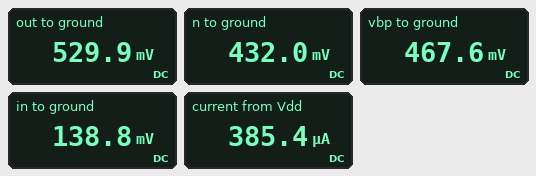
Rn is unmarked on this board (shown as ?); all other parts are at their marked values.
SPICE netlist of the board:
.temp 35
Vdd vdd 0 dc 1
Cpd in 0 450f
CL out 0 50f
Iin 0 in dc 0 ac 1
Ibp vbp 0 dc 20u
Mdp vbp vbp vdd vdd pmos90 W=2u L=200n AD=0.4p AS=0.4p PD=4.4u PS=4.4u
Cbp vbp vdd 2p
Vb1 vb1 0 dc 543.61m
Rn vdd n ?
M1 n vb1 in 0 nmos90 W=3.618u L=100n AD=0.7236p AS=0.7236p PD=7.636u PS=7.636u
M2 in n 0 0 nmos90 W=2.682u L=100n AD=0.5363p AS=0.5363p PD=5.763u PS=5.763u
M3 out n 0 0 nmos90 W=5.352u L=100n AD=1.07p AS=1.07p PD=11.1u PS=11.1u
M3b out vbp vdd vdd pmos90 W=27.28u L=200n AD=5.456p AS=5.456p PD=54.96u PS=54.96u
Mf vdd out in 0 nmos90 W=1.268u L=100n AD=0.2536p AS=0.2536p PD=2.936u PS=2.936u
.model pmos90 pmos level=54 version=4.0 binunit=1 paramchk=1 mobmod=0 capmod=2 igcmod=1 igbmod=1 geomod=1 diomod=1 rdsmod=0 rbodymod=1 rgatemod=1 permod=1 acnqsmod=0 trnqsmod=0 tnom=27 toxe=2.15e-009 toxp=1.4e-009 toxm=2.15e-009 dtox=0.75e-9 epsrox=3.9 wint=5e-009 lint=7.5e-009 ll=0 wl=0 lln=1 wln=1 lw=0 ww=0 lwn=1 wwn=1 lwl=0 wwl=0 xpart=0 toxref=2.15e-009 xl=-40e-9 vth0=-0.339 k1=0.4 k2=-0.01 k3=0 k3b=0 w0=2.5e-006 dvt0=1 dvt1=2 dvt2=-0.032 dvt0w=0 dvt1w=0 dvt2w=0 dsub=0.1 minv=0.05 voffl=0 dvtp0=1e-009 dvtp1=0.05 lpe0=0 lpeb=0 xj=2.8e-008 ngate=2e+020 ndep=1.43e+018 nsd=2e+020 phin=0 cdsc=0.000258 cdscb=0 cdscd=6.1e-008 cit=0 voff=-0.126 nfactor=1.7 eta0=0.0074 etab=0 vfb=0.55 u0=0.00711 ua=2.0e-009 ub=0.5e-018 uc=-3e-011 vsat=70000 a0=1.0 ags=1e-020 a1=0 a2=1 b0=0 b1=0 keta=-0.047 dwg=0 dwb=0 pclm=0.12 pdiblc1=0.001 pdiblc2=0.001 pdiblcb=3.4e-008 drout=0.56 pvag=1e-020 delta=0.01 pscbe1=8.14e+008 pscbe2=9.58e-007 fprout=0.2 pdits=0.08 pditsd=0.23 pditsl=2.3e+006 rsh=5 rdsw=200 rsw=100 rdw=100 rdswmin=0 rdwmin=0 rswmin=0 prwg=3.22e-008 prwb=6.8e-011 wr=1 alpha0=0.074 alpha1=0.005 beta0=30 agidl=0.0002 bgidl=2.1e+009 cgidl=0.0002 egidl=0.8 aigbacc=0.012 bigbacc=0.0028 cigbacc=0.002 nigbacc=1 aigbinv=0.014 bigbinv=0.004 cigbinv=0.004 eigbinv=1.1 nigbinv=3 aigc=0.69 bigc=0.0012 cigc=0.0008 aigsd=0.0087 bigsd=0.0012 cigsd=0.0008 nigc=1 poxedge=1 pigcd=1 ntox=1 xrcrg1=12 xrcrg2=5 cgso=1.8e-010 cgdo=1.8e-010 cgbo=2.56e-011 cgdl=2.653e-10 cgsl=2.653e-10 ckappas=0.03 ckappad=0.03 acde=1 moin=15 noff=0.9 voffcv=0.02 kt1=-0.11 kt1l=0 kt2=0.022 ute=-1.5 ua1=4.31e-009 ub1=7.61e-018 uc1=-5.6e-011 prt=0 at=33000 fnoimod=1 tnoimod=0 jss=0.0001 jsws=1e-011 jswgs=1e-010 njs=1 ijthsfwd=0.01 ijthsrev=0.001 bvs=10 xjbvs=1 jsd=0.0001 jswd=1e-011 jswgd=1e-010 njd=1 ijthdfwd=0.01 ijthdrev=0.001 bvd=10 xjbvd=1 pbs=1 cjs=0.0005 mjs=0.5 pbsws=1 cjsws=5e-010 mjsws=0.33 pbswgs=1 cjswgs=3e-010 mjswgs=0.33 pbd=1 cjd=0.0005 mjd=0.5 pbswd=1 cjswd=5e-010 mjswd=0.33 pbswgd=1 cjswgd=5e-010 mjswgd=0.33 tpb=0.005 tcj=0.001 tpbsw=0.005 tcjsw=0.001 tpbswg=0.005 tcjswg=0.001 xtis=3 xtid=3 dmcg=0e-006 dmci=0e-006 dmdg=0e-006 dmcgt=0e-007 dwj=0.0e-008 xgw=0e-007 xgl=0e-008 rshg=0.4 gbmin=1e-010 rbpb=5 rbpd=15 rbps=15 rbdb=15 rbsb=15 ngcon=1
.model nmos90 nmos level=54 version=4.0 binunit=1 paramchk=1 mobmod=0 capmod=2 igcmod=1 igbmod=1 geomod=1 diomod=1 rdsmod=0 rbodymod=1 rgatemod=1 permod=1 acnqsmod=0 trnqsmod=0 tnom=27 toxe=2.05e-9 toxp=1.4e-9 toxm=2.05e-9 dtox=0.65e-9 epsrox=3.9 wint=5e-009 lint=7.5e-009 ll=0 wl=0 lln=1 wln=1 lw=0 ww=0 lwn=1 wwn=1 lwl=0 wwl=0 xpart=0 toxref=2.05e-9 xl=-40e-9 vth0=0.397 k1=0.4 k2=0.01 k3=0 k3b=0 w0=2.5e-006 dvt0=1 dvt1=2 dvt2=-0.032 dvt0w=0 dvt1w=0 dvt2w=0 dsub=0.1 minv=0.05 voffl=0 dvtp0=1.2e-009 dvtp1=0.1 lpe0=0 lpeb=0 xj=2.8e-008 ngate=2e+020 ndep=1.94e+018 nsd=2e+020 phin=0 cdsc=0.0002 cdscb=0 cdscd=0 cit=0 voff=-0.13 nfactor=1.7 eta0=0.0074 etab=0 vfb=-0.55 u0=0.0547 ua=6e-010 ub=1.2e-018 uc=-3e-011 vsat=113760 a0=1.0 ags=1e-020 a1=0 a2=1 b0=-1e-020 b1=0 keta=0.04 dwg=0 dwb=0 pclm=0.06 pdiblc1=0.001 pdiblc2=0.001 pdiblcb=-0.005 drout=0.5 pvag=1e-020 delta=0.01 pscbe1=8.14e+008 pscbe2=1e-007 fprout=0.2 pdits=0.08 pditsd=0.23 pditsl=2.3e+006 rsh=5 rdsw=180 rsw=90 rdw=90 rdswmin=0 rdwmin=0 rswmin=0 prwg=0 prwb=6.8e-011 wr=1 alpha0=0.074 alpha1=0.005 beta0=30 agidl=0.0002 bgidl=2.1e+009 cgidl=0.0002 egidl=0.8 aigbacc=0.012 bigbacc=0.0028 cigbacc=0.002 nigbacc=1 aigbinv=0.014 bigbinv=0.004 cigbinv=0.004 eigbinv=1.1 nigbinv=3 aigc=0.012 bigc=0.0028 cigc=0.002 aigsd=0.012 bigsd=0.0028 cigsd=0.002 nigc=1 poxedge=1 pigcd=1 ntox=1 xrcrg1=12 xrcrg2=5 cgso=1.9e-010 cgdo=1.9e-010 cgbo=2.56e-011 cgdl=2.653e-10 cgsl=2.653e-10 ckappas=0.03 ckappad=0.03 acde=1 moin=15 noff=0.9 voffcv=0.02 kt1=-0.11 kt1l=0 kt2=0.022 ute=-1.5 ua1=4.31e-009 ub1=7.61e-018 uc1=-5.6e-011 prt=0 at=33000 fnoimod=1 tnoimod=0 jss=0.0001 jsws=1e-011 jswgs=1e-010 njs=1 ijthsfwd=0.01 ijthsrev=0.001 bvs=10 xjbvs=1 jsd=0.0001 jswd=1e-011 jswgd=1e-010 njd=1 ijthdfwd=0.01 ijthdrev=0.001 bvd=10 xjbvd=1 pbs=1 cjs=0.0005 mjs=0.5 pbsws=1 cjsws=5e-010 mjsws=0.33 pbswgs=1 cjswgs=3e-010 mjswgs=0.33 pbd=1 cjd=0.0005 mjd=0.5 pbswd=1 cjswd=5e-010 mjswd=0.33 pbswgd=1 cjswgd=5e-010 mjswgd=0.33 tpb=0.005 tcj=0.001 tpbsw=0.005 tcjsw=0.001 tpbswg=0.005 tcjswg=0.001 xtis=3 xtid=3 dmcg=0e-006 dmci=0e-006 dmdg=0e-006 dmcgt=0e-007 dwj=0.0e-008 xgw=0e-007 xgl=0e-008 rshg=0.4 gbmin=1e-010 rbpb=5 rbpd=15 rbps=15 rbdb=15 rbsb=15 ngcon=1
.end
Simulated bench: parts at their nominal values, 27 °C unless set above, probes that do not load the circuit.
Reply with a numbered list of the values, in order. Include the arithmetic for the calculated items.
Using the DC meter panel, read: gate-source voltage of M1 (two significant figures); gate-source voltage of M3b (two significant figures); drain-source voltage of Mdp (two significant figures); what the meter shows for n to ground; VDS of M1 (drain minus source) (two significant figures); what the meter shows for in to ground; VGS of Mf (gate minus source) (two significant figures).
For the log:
1. 543.6 mV - 138.8 mV = 400 mV
2. 467.6 mV - 1 V = -530 mV
3. 467.6 mV - 1 V = -530 mV
4. 432.0 mV
5. 432 mV - 138.8 mV = 290 mV
6. 138.8 mV
7. 529.9 mV - 138.8 mV = 390 mV
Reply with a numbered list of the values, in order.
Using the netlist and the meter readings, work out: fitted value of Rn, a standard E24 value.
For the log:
1. 9.1 kΩ
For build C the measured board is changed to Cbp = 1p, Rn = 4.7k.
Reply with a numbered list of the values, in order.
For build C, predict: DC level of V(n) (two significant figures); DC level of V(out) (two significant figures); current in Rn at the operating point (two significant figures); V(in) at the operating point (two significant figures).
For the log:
1. 450 mV
2. 250 mV
3. 120 µA
4. 110 mV
